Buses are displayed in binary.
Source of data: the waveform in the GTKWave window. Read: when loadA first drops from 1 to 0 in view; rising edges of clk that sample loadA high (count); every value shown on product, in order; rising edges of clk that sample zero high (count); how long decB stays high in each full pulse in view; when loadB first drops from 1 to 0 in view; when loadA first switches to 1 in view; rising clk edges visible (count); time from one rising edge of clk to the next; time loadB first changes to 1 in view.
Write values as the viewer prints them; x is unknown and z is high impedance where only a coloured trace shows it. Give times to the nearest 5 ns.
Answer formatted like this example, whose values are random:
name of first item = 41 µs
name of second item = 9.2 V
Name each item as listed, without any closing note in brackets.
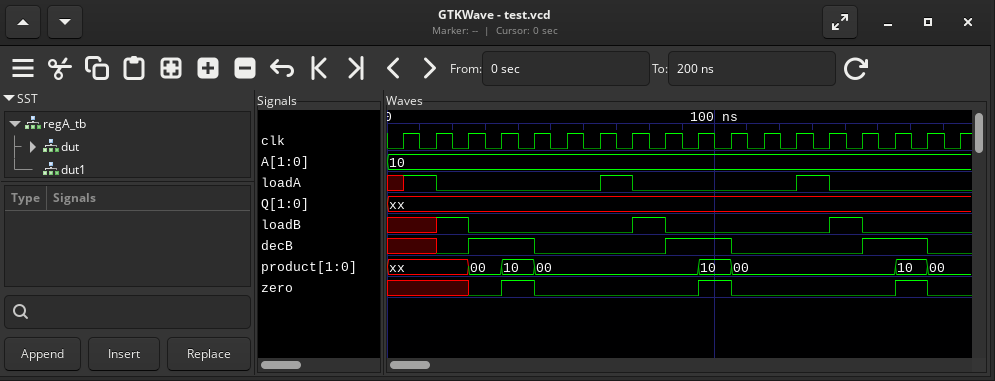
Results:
when loadA first drops from 1 to 0 in view = 15 ns
rising edges of clk that sample loadA high = 3
every value shown on product, in order = xx, 00, 10, 00, 10, 00, 10, 00
rising edges of clk that sample zero high = 3
how long decB stays high in each full pulse in view = 20 ns, 20 ns, 20 ns
when loadB first drops from 1 to 0 in view = 25 ns
when loadA first switches to 1 in view = 5 ns
rising clk edges visible = 18
time from one rising edge of clk to the next = 10 ns
time loadB first changes to 1 in view = 15 ns
